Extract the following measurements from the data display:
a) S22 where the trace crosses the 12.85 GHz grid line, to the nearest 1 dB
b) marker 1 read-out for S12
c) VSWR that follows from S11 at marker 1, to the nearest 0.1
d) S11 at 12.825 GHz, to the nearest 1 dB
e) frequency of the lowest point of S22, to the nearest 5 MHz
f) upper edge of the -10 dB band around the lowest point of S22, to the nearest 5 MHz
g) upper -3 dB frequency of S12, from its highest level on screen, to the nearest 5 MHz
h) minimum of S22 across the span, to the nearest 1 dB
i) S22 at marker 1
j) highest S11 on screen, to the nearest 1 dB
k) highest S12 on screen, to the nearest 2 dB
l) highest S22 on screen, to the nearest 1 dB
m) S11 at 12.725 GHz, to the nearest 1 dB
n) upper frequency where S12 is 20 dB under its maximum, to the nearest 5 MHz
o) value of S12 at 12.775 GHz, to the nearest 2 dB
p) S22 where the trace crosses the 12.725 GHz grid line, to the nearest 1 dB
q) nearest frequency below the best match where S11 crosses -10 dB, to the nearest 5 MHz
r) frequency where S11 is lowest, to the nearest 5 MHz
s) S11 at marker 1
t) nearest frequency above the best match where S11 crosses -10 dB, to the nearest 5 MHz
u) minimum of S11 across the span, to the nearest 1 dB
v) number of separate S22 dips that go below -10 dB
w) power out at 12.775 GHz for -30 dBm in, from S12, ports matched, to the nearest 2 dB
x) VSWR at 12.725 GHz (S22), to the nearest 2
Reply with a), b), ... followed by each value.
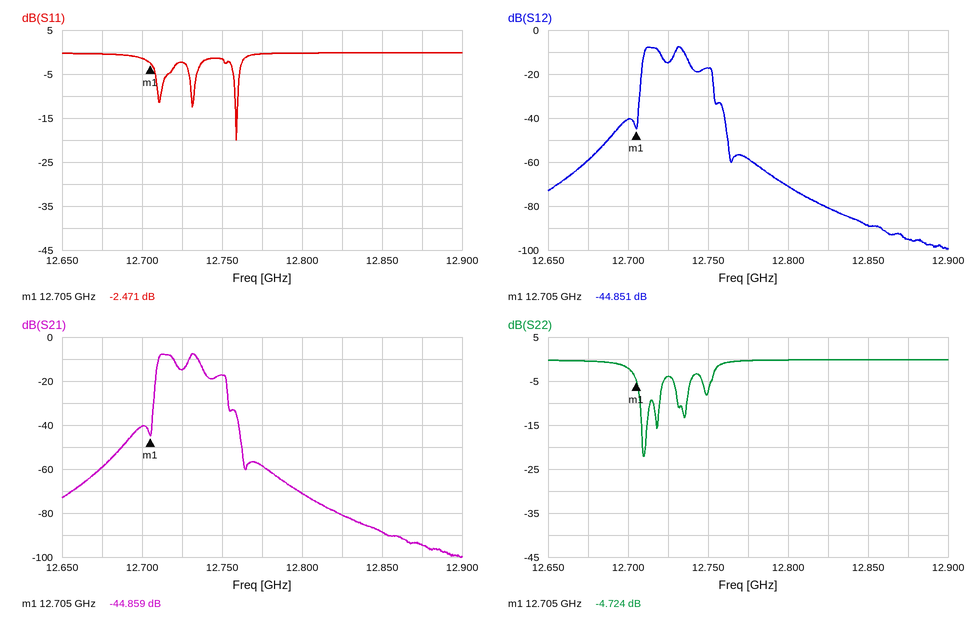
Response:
a) 0 dB
b) -44.851 dB
c) 7.1
d) 0 dB
e) 12.710 GHz
f) 12.715 GHz
g) 12.735 GHz
h) -22 dB
i) -4.724 dB
j) 0 dB
k) -8 dB
l) 0 dB
m) -2 dB
n) 12.755 GHz
o) -58 dB
p) -4 dB
q) 12.760 GHz
r) 12.760 GHz
s) -2.471 dB
t) 12.760 GHz
u) -20 dB
v) 3
w) -88 dBm
x) 4
